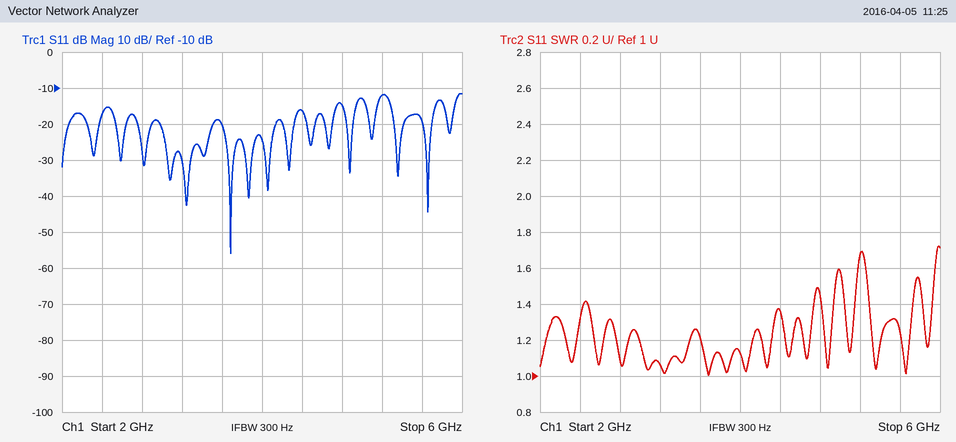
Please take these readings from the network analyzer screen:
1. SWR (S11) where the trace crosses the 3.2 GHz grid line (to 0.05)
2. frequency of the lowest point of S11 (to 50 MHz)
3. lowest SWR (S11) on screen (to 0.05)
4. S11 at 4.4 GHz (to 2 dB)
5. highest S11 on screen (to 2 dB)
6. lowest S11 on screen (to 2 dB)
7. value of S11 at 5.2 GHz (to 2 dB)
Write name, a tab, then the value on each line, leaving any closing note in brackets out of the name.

SWR (S11) where the trace crosses the 3.2 GHz grid line	1.05
frequency of the lowest point of S11	3.70 GHz
lowest SWR (S11) on screen	1.00
S11 at 4.4 GHz	-16 dB
highest S11 on screen	-12 dB
lowest S11 on screen	-56 dB
value of S11 at 5.2 GHz	-12 dB
